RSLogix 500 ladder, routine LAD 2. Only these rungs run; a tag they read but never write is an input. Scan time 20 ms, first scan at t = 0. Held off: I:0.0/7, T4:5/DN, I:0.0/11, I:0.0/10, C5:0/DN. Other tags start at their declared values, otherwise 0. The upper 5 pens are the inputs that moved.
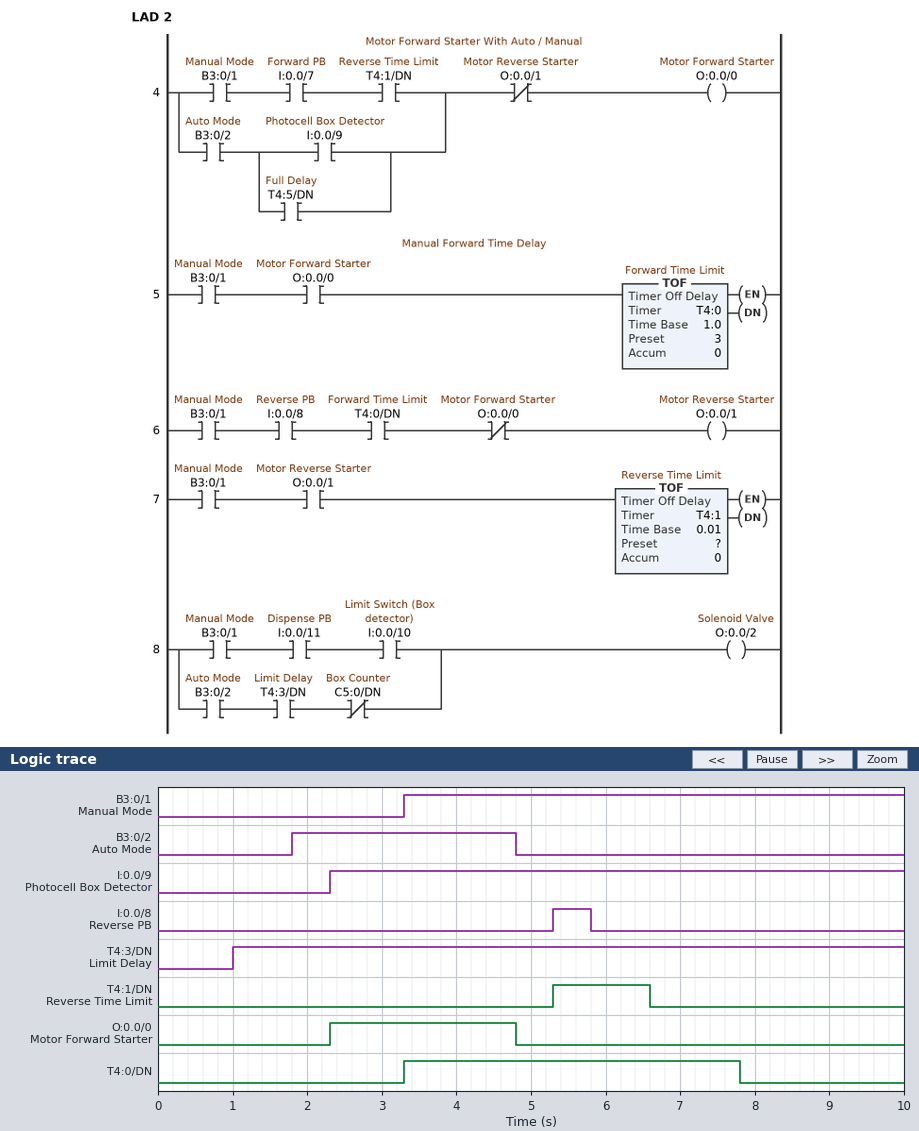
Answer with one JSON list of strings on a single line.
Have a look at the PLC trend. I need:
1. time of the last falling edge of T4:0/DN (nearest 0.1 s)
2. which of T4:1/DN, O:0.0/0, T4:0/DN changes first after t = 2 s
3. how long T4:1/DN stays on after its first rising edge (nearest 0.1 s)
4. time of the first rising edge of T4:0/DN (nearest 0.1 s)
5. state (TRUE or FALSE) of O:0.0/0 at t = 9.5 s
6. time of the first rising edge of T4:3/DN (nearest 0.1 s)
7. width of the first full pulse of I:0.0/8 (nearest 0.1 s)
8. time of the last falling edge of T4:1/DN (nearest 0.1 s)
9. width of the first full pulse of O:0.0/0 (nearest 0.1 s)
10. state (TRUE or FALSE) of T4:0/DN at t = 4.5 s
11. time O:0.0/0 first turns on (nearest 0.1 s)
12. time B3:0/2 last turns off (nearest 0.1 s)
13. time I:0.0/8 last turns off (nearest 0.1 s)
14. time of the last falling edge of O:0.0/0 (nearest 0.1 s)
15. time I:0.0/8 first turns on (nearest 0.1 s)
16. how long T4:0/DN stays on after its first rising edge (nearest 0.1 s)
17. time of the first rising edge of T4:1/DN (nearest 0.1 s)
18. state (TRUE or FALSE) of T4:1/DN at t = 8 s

["7.8 s", "O:0.0/0", "1.3 s", "3.3 s", "FALSE", "1.0 s", "0.5 s", "6.6 s", "2.5 s", "TRUE", "2.3 s", "4.8 s", "5.8 s", "4.8 s", "5.3 s", "4.5 s", "5.3 s", "FALSE"]
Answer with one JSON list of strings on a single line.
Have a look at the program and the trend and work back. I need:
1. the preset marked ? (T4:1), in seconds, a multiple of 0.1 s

["0.8 s"]
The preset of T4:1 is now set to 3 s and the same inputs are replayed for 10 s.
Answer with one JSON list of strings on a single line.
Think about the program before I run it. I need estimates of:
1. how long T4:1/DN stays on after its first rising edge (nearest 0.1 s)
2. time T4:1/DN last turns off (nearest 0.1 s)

["3.5 s", "8.8 s"]
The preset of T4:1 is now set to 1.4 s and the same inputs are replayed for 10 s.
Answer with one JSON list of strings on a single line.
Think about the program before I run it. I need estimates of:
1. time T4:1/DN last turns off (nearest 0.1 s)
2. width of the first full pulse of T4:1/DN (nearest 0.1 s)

["7.2 s", "1.9 s"]
